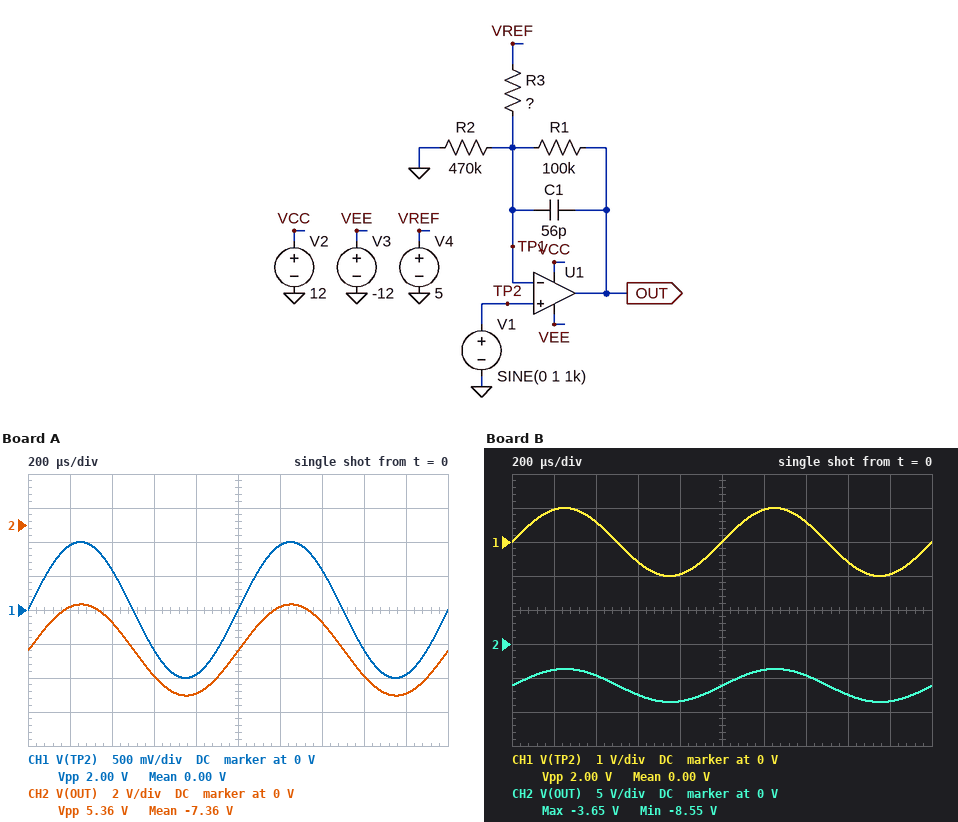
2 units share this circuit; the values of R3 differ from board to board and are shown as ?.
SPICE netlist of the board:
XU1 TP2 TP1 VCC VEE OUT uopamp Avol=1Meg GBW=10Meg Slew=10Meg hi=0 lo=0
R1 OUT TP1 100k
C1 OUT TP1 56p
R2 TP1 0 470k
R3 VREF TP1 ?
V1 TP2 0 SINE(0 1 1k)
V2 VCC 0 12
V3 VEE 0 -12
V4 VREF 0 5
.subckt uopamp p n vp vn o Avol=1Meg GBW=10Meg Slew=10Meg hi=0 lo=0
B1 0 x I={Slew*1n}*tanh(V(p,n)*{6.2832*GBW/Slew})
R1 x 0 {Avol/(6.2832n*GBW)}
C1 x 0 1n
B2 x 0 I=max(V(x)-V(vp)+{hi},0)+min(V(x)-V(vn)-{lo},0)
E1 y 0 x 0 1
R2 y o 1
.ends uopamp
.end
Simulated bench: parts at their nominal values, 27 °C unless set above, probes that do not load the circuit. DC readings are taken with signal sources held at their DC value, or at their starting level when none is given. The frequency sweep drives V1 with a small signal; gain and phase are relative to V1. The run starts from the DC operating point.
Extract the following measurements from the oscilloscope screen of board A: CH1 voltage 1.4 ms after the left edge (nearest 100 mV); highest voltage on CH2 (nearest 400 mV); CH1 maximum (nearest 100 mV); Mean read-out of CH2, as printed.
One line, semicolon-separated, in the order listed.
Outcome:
600 mV; -4.8 V; 1.0 V; -7.36 V
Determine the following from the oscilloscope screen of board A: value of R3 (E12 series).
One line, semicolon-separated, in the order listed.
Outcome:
68 kΩ
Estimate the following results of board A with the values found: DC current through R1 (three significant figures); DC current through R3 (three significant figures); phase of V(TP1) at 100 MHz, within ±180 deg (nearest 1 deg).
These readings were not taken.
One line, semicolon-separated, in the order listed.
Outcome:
73.5 µA; 73.5 µA; -84 deg
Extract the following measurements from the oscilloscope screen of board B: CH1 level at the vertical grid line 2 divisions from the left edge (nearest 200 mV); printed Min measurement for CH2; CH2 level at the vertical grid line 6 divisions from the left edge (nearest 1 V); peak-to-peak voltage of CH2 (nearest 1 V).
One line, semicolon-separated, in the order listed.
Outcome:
600 mV; -8.55 V; -4 V; 5 V
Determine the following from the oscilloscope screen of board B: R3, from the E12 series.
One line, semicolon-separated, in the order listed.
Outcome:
82 kΩ
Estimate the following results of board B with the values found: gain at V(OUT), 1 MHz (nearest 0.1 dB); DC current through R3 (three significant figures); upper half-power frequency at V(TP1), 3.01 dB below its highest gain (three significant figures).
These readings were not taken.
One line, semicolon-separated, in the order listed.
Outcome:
-0.1 dB; 61.0 µA; 9.96 MHz
